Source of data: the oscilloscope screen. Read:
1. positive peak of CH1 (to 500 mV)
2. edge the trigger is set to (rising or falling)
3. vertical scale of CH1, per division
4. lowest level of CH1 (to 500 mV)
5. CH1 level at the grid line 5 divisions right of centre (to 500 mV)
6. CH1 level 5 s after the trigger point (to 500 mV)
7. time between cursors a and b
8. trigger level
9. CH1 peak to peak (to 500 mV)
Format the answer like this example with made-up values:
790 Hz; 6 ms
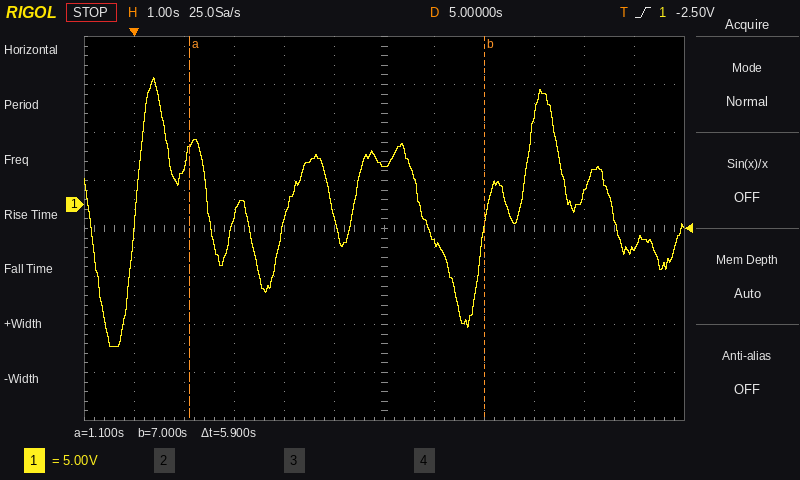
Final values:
13.0 V; rising; 5 V; -15.0 V; -4.5 V; 4.0 V; 5.9 s; -2.50 V; 28.0 V
